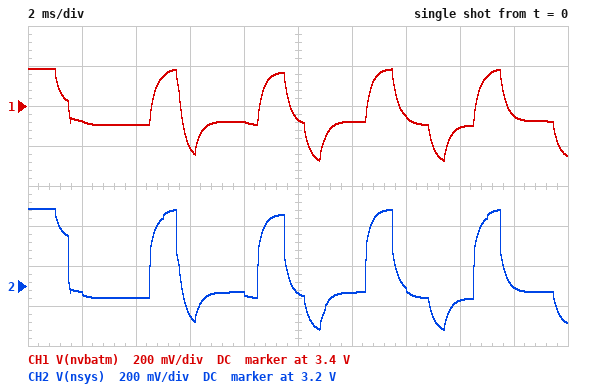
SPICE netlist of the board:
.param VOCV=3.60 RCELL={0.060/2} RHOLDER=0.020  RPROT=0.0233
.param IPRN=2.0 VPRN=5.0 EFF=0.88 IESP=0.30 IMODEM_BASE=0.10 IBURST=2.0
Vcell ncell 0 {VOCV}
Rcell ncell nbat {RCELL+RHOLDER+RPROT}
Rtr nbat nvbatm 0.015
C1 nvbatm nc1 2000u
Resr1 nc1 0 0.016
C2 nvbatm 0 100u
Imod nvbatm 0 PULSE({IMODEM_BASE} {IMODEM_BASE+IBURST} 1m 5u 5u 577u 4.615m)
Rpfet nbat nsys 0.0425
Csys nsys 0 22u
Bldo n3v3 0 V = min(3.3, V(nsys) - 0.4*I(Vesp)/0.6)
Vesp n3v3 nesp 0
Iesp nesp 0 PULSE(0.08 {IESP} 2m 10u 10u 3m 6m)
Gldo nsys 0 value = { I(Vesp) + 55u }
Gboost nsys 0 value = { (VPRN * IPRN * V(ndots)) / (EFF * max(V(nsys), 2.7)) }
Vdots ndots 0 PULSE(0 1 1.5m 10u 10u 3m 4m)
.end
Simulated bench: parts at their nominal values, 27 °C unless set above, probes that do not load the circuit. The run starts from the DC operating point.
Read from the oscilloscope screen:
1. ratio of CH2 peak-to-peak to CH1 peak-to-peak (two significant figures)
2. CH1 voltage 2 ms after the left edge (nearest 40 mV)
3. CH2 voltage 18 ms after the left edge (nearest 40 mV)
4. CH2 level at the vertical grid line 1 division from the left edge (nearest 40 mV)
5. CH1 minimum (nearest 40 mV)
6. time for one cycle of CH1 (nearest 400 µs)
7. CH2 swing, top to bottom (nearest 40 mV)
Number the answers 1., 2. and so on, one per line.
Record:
1. 1.3
2. 3.32 V
3. 3.20 V
4. 3.16 V
5. 3.12 V
6. 4.0 ms
7. 600 mV
